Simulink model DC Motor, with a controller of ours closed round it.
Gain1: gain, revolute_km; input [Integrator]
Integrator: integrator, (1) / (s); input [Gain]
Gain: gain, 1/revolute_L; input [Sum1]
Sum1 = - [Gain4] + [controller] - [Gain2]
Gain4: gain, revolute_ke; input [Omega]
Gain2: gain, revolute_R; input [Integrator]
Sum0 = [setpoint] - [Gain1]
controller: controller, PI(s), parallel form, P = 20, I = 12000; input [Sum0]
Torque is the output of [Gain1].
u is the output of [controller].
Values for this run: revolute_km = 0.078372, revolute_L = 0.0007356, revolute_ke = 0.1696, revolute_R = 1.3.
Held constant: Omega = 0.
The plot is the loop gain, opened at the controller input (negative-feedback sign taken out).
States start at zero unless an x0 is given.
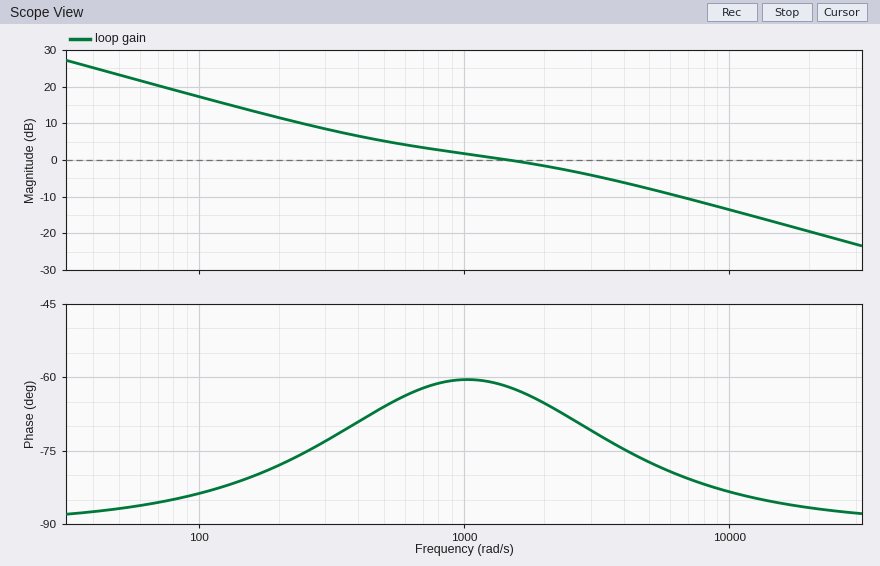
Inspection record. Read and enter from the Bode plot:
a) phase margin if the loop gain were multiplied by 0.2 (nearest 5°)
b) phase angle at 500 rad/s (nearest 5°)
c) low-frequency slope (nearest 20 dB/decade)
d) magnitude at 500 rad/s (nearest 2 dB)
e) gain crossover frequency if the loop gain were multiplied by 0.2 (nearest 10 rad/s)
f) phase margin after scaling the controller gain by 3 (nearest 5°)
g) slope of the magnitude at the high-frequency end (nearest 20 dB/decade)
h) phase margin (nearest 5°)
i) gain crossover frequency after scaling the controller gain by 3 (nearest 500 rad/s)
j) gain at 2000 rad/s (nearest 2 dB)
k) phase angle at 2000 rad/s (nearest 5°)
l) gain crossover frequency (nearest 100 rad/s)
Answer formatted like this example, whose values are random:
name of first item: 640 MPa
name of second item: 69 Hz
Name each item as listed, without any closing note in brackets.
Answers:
phase margin if the loop gain were multiplied by 0.2: 100°
phase angle at 500 rad/s: -65°
low-frequency slope: -20 dB/decade
magnitude at 500 rad/s: 6 dB
gain crossover frequency if the loop gain were multiplied by 0.2: 150 rad/s
phase margin after scaling the controller gain by 3: 100°
slope of the magnitude at the high-frequency end: -20 dB/decade
phase margin: 120°
gain crossover frequency after scaling the controller gain by 3: 6000 rad/s
gain at 2000 rad/s: -2 dB
phase angle at 2000 rad/s: -65°
gain crossover frequency: 1500 rad/s
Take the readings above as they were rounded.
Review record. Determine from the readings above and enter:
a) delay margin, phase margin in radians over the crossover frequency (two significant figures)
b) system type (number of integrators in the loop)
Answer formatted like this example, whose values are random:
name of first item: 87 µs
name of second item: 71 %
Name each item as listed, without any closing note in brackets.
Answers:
delay margin, phase margin in radians over the crossover frequency: 0.0014 s
system type: 1
